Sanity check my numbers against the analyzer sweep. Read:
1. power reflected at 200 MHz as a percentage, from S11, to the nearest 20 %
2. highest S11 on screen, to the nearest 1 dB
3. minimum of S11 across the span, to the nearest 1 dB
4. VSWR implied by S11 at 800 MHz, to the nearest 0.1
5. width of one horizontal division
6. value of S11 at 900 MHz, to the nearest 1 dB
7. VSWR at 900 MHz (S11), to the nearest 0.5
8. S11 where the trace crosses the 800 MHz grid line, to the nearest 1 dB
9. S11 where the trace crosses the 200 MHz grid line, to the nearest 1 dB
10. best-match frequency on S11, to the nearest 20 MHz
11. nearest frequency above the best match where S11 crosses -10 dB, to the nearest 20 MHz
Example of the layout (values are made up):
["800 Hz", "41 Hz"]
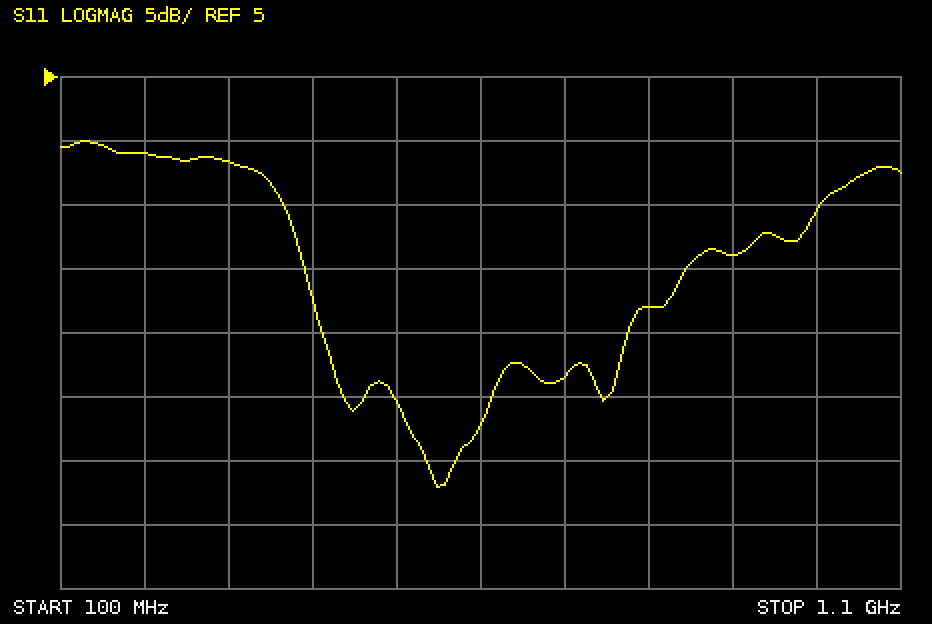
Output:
["80 %", "0 dB", "-27 dB", "1.6", "100 MHz", "-9 dB", "2.0", "-13 dB", "-1 dB", "540 MHz", "840 MHz"]
